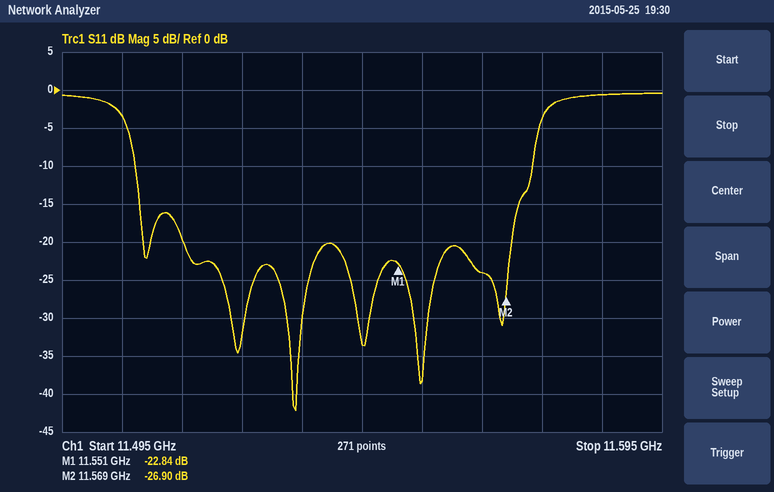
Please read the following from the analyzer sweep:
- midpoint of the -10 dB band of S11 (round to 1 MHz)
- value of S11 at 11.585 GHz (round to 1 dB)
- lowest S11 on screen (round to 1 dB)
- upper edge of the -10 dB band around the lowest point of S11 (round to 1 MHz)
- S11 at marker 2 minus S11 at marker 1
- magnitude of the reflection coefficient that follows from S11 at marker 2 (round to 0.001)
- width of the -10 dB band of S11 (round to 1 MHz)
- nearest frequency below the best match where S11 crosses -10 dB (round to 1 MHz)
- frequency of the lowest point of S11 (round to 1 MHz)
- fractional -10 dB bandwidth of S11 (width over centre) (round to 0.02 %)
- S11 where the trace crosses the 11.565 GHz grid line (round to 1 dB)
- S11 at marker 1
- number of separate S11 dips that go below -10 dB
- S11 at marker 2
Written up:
11.540 GHz
-1 dB
-42 dB
11.573 GHz
-4.06 dB
0.045
66 MHz
11.507 GHz
11.534 GHz
0.58 %
-24 dB
-22.84 dB
6
-26.90 dB
